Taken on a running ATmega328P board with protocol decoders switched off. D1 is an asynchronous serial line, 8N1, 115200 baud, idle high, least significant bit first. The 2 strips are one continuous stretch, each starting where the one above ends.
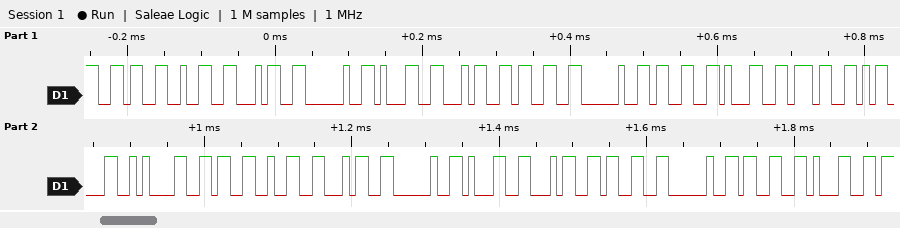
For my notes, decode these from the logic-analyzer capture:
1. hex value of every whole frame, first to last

0x36 0x32 0x34 0x20 0x31 0x34 0x33 0x20 0x33 0x31 0x37 0x0D 0x0A 0x36 0x32 0x34 0x20 0x31 0x34 0x33 0x20 0x33 0x31
